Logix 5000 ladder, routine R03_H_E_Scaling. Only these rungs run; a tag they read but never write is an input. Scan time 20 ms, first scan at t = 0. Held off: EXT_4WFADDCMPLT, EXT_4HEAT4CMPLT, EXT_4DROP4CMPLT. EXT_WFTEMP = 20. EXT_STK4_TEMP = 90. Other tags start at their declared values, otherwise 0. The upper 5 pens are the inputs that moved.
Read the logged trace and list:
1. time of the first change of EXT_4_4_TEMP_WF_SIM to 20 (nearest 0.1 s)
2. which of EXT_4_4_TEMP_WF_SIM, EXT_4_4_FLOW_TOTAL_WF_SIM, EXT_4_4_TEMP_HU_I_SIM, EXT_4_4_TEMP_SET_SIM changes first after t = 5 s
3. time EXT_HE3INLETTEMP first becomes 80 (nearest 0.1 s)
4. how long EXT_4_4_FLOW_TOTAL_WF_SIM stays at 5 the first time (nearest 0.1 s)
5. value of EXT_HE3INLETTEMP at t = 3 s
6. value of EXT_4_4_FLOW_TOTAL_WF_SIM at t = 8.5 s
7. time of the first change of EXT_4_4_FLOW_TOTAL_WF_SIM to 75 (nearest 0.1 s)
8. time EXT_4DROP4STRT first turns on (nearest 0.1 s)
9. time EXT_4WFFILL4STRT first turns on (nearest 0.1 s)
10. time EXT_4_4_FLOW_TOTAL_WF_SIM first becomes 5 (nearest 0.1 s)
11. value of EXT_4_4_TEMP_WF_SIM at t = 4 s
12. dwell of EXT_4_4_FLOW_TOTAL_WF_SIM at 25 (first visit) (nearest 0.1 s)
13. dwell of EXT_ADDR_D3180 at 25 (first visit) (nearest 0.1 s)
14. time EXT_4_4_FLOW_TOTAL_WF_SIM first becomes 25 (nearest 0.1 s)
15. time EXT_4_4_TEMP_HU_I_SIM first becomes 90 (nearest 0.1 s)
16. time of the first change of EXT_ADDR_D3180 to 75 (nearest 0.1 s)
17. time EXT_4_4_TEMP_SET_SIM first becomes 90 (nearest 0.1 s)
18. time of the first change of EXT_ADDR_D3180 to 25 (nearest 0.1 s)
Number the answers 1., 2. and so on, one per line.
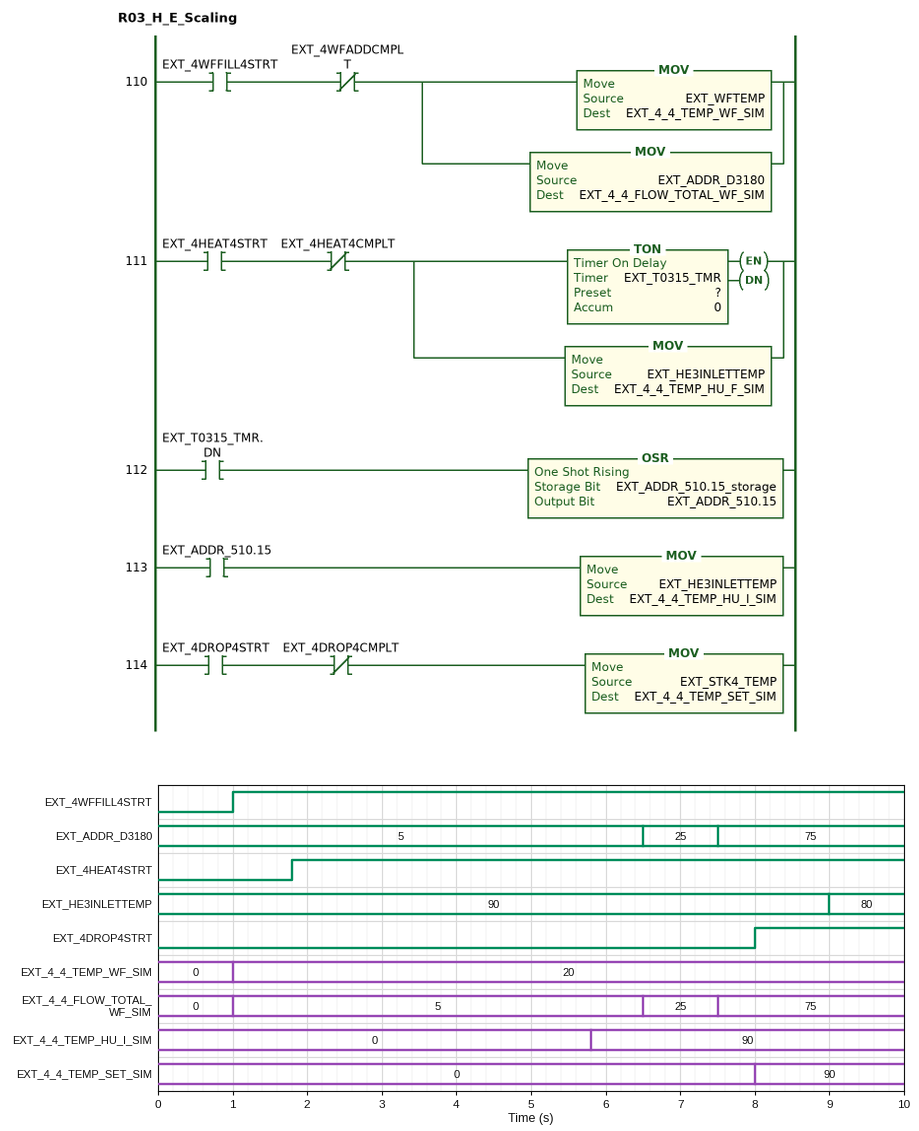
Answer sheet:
1. 1.0 s
2. EXT_4_4_TEMP_HU_I_SIM
3. 9.0 s
4. 5.5 s
5. 90
6. 75
7. 7.5 s
8. 8.0 s
9. 1.0 s
10. 1.0 s
11. 20
12. 1.0 s
13. 1.0 s
14. 6.5 s
15. 5.8 s
16. 7.5 s
17. 8.0 s
18. 6.5 s
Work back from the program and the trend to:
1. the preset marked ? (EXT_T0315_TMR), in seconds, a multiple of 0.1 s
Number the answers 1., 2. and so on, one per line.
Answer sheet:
1. 4.0 s
